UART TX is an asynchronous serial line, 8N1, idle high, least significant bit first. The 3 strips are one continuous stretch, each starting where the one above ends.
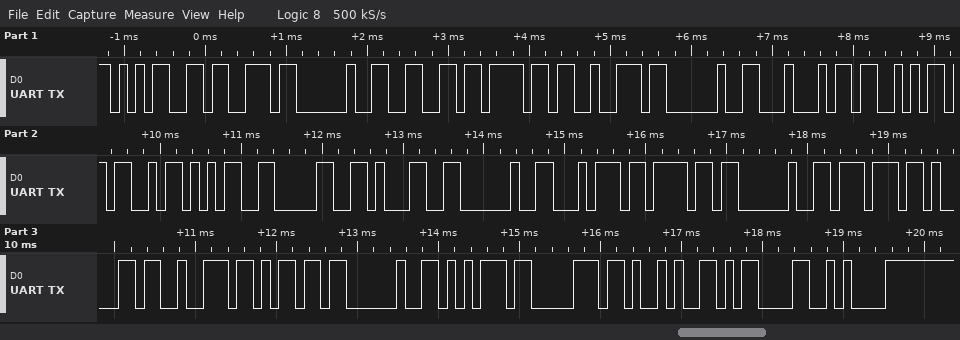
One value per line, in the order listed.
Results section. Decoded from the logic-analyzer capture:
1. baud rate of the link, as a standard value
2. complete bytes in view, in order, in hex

9600 baud
0x35 0x73 0x20 0x66 0x6F 0x72 0x20 0x44 0x53 0x4D 0x35 0x30 0x31 0x20 0x74 0x6F 0x20 0x77 0x61 0x72 0x6D 0x20 0x75 0x70 0x29 0x0D 0x0A
